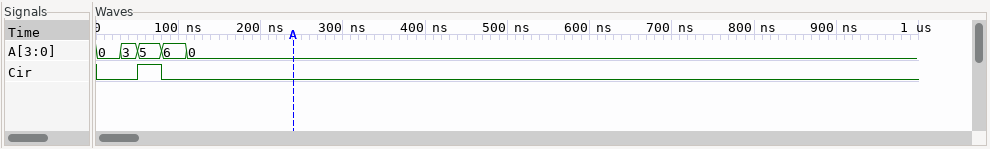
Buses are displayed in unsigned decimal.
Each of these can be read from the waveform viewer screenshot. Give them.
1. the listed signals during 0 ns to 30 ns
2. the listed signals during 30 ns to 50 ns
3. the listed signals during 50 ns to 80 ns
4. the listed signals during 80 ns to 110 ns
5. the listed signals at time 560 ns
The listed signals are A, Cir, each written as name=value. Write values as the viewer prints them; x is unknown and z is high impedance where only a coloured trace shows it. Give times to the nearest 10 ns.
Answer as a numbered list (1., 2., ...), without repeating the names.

1. A=0, Cir=0
2. A=3, Cir=0
3. A=5, Cir=1
4. A=6, Cir=0
5. A=0, Cir=0
